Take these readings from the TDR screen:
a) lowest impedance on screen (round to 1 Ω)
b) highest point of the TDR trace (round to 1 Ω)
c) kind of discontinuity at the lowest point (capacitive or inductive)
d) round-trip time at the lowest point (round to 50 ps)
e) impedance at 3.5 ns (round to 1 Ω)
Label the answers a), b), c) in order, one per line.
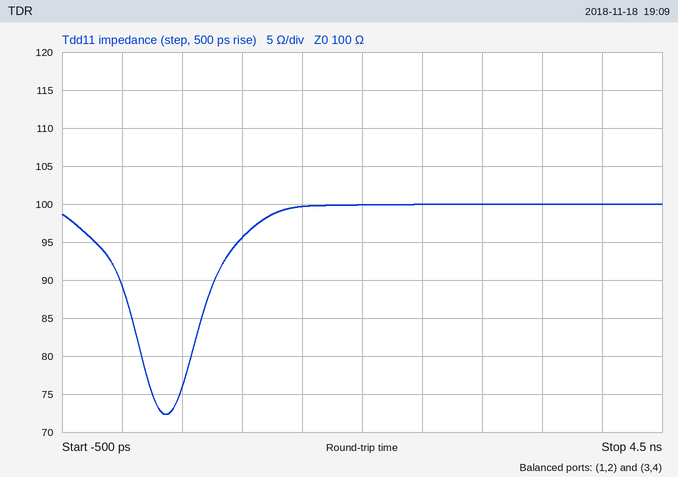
a) 72 Ω
b) 100 Ω
c) capacitive
d) 350 ps
e) 100 Ω
